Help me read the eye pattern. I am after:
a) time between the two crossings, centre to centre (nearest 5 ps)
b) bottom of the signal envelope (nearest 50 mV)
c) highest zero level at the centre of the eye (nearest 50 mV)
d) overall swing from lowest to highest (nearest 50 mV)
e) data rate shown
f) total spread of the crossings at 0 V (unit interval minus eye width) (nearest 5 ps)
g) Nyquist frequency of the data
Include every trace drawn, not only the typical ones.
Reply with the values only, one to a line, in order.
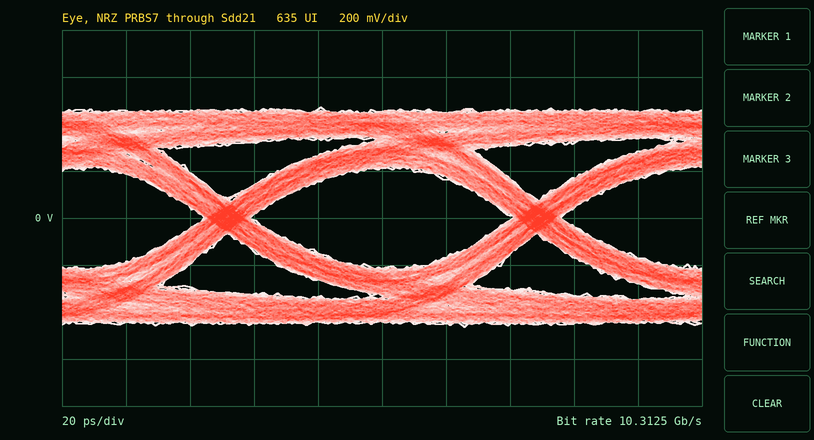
95 ps
-450 mV
-200 mV
950 mV
10.3125 Gb/s
15 ps
5.15625 GHz
